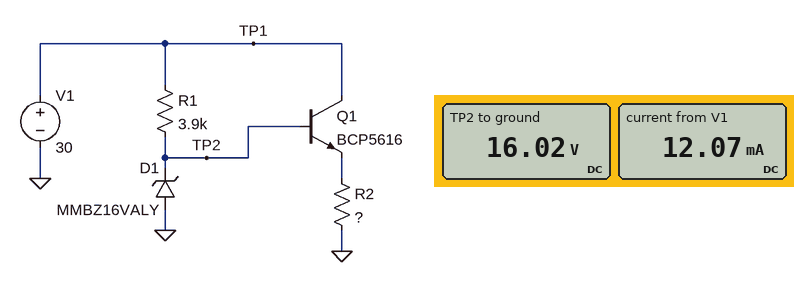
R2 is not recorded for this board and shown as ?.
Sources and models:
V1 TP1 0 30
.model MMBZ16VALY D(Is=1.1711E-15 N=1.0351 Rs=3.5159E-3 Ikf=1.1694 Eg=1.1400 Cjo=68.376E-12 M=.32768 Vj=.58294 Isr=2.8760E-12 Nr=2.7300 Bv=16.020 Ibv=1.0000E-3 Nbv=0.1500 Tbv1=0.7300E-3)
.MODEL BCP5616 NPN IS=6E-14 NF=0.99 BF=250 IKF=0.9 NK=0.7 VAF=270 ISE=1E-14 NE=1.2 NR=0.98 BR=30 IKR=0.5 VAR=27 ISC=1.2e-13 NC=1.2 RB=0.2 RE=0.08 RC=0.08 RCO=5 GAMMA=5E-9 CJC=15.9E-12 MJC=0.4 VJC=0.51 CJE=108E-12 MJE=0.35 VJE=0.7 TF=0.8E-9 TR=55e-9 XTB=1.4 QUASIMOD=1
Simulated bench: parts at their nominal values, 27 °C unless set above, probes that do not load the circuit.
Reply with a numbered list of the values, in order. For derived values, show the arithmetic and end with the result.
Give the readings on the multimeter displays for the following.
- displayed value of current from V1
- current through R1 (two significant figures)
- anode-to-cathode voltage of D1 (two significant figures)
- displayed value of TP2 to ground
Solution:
1. 12.07 mA
2. (30 V - 16.02 V) / 3.9 kΩ = 3.6 mA
3. 0 V - 16.02 V = -16 V
4. 16.02 V
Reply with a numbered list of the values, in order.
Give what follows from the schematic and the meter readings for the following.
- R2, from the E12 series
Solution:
1. 1.8 kΩ
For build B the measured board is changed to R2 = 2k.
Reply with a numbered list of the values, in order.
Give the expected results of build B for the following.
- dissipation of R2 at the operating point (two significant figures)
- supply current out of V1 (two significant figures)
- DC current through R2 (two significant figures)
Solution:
1. 120 mW
2. 11 mA
3. 7.7 mA
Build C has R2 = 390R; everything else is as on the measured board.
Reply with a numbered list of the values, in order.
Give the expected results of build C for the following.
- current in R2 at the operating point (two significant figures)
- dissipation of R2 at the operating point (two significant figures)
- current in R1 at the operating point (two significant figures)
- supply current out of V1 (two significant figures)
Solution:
1. 39 mA
2. 600 mW
3. 3.6 mA
4. 43 mA
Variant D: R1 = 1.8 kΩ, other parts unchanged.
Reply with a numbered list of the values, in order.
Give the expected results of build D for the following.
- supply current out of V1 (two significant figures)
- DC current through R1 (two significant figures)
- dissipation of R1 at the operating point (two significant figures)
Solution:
1. 16 mA
2. 7.8 mA
3. 110 mW
